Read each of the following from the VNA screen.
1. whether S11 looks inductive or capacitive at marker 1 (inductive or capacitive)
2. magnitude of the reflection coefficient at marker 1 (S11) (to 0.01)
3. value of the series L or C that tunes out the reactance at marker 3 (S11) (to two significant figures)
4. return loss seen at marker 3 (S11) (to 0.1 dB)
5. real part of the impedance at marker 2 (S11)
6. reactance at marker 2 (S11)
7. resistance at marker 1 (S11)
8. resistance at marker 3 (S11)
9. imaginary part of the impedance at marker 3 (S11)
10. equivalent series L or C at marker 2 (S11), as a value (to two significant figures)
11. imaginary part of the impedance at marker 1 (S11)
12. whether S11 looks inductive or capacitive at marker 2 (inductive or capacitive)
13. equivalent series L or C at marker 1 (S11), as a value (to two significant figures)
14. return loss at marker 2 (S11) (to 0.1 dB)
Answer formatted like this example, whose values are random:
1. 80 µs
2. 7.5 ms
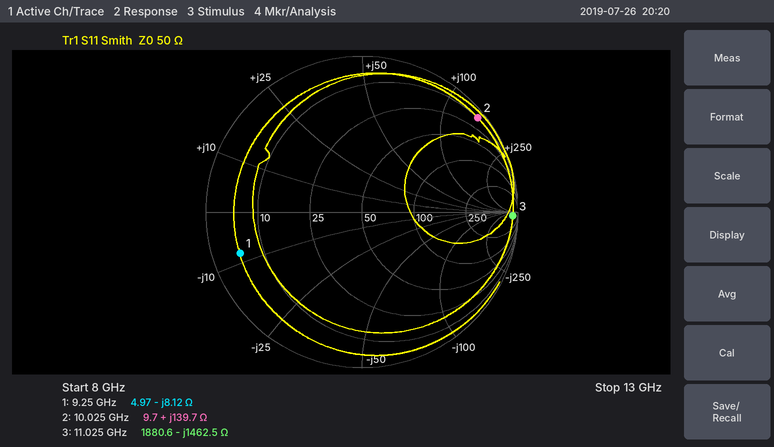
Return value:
1. capacitive
2. 0.82
3. 21 nH
4. 0.3 dB
5. 9.7 Ω
6. +139.7 Ω
7. 4.97 Ω
8. 1880.6 Ω
9. -1462.5 Ω
10. 2.2 nH
11. -8.12 Ω
12. inductive
13. 2.1 pF
14. 0.4 dB
